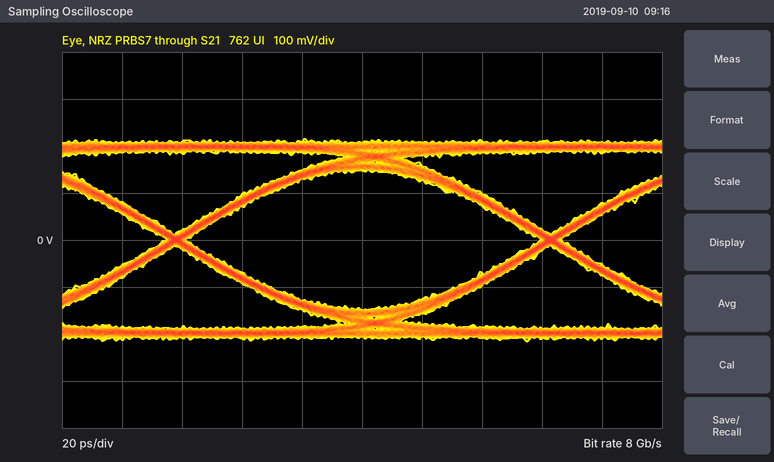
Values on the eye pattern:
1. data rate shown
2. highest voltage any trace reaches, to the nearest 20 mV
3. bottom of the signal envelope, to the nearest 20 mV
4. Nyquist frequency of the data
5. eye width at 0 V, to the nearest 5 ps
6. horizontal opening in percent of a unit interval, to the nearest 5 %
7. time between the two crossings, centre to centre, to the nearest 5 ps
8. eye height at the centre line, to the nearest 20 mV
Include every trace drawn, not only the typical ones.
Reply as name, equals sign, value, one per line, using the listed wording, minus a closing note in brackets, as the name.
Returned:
data rate shown = 8 Gb/s
highest voltage any trace reaches, to the nearest 20 mV = 220 mV
bottom of the signal envelope, to the nearest 20 mV = -220 mV
Nyquist frequency of the data = 4 GHz
eye width at 0 V, to the nearest 5 ps = 120 ps
horizontal opening in percent of a unit interval, to the nearest 5 % = 95 %
time between the two crossings, centre to centre, to the nearest 5 ps = 125 ps
eye height at the centre line, to the nearest 20 mV = 300 mV
